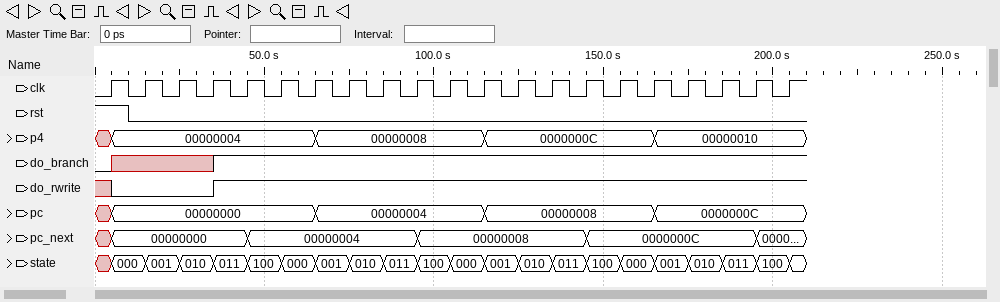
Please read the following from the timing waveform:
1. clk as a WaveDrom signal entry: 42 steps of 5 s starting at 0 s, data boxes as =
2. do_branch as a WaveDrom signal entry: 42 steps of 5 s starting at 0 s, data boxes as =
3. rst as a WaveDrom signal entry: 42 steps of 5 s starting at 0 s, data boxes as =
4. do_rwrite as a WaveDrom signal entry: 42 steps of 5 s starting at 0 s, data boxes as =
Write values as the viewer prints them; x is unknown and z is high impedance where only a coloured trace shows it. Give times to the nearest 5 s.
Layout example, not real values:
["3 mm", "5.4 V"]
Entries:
["{name: 'clk', wave: '010101010101010101010101010101010101010101'}", "{name: 'do_branch', wave: '0x.....1..................................'}", "{name: 'rst', wave: '1.0.......................................'}", "{name: 'do_rwrite', wave: 'x0.....1..................................'}"]
